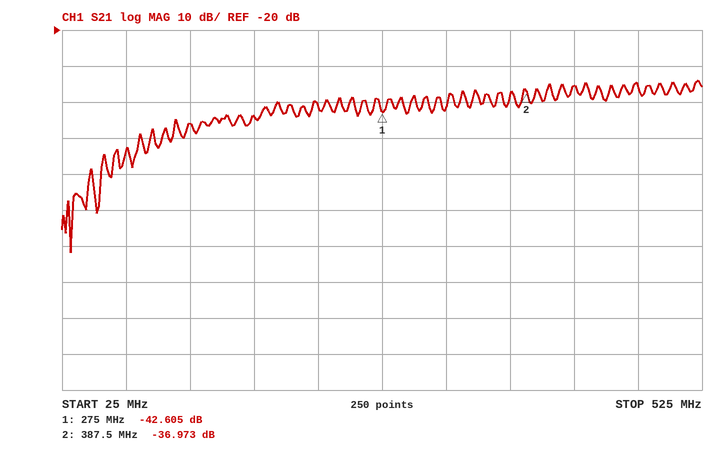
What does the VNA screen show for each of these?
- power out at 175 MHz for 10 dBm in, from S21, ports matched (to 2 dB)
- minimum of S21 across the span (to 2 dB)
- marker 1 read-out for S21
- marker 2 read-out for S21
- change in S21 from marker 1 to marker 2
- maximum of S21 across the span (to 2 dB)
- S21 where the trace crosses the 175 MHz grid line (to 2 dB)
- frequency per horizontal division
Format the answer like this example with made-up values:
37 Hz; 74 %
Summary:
-34 dBm; -82 dB; -42.605 dB; -36.973 dB; 5.632 dB; -34 dB; -44 dB; 50 MHz
